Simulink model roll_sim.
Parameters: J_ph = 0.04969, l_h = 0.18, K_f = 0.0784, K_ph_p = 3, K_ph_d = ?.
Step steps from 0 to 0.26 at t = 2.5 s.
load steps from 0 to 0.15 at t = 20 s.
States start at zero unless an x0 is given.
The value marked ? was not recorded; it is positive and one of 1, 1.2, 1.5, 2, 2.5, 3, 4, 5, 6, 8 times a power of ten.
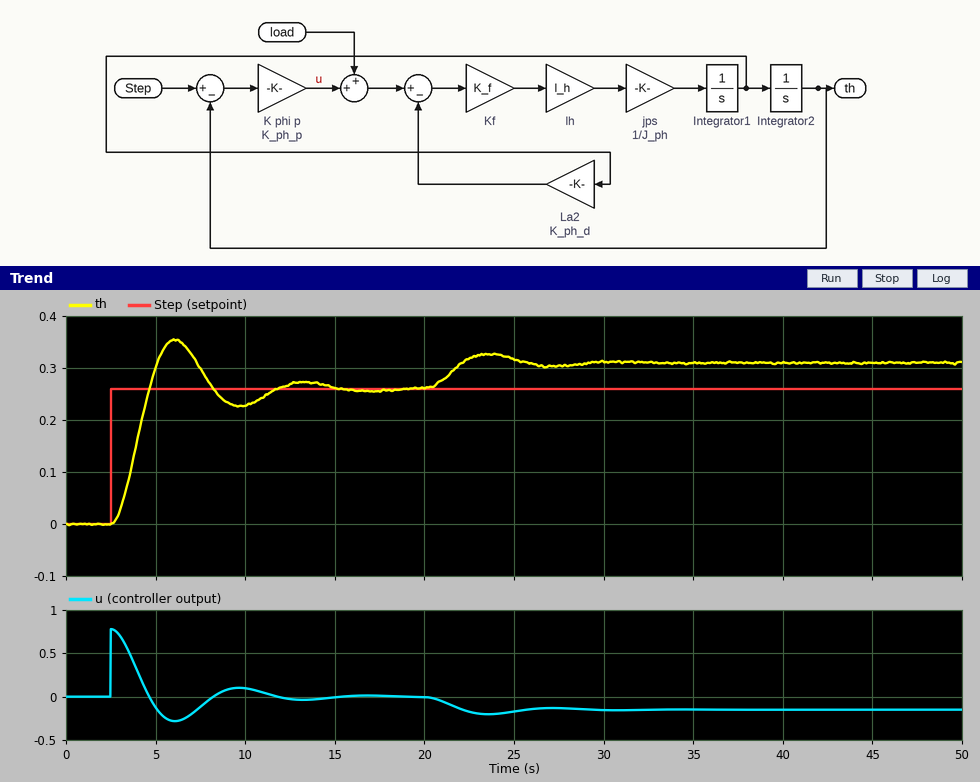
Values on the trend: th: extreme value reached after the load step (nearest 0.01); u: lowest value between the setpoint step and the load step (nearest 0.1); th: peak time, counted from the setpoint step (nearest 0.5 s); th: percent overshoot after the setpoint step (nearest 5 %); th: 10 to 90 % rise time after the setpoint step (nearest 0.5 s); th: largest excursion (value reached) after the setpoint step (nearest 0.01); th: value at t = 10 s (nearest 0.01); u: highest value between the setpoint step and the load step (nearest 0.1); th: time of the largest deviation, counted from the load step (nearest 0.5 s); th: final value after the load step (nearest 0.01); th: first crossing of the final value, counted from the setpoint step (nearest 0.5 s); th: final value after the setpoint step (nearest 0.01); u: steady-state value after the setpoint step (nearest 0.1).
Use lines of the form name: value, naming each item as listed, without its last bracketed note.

th: extreme value reached after the load step: 0.33
u: lowest value between the setpoint step and the load step: -0.3
th: peak time, counted from the setpoint step: 3.5 s
th: percent overshoot after the setpoint step: 35 %
th: 10 to 90 % rise time after the setpoint step: 1.5 s
th: largest excursion (value reached) after the setpoint step: 0.35
th: value at t = 10 s: 0.23
u: highest value between the setpoint step and the load step: 0.8
th: time of the largest deviation, counted from the load step: 3.5 s
th: final value after the load step: 0.31
th: first crossing of the final value, counted from the setpoint step: 2.0 s
th: final value after the setpoint step: 0.26
u: steady-state value after the setpoint step: 0.0
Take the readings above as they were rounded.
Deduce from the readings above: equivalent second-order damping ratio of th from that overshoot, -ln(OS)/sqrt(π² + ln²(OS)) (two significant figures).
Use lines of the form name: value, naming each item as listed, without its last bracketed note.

equivalent second-order damping ratio of th from that overshoot, -ln(OS)/sqrt(π² + ln²(OS)): 0.32
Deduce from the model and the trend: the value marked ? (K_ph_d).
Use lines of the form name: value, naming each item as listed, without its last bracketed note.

the value marked ?: 2
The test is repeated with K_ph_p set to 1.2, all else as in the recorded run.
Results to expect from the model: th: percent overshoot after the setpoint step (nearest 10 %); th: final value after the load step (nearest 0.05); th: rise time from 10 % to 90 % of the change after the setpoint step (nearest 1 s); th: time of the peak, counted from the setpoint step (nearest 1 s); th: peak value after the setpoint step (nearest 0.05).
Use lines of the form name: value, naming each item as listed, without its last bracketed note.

th: percent overshoot after the setpoint step: 20 %
th: final value after the load step: 0.40
th: rise time from 10 % to 90 % of the change after the setpoint step: 3 s
th: time of the peak, counted from the setpoint step: 6 s
th: peak value after the setpoint step: 0.30
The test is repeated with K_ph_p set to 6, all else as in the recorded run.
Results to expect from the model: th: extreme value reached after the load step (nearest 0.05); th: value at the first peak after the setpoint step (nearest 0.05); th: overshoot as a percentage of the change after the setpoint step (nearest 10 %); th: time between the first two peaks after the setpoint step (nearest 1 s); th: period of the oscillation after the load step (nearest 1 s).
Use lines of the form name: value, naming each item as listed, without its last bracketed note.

th: extreme value reached after the load step: 0.30
th: value at the first peak after the setpoint step: 0.40
th: overshoot as a percentage of the change after the setpoint step: 50 %
th: time between the first two peaks after the setpoint step: 5 s
th: period of the oscillation after the load step: 5 s
